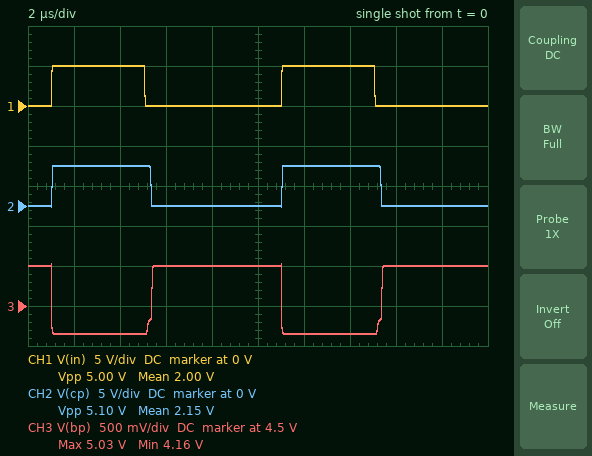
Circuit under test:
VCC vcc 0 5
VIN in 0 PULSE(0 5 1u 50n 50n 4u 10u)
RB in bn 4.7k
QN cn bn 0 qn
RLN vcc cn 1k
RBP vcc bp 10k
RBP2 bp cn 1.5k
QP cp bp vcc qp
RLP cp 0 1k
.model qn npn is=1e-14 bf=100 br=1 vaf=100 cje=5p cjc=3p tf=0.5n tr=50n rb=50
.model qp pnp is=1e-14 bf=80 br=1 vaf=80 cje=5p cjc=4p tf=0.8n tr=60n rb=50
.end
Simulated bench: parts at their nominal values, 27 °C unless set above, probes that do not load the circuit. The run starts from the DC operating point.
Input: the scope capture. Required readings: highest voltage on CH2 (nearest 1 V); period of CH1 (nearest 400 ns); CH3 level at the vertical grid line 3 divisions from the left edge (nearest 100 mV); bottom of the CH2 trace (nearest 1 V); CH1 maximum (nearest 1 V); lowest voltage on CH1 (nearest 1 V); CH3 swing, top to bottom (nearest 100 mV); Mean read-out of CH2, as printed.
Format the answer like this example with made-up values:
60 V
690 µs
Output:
5 V
10.0 µs
5.0 V
0 V
5 V
0 V
900 mV
2.15 V
